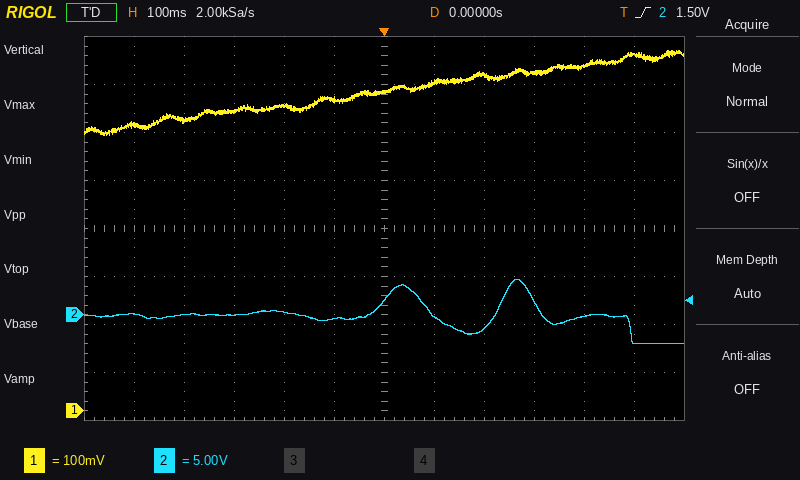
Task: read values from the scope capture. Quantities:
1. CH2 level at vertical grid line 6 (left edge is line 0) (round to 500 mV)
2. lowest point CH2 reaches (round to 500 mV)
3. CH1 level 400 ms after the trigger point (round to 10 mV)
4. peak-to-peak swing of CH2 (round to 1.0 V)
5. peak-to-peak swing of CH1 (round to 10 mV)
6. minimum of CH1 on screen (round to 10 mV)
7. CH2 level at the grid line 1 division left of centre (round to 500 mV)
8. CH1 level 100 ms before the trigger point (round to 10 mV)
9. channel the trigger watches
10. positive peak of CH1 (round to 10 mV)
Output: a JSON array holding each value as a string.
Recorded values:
["1.5 V", "-3.0 V", "720 mV", "7.0 V", "180 mV", "570 mV", "-500 mV", "650 mV", "CH2", "750 mV"]
